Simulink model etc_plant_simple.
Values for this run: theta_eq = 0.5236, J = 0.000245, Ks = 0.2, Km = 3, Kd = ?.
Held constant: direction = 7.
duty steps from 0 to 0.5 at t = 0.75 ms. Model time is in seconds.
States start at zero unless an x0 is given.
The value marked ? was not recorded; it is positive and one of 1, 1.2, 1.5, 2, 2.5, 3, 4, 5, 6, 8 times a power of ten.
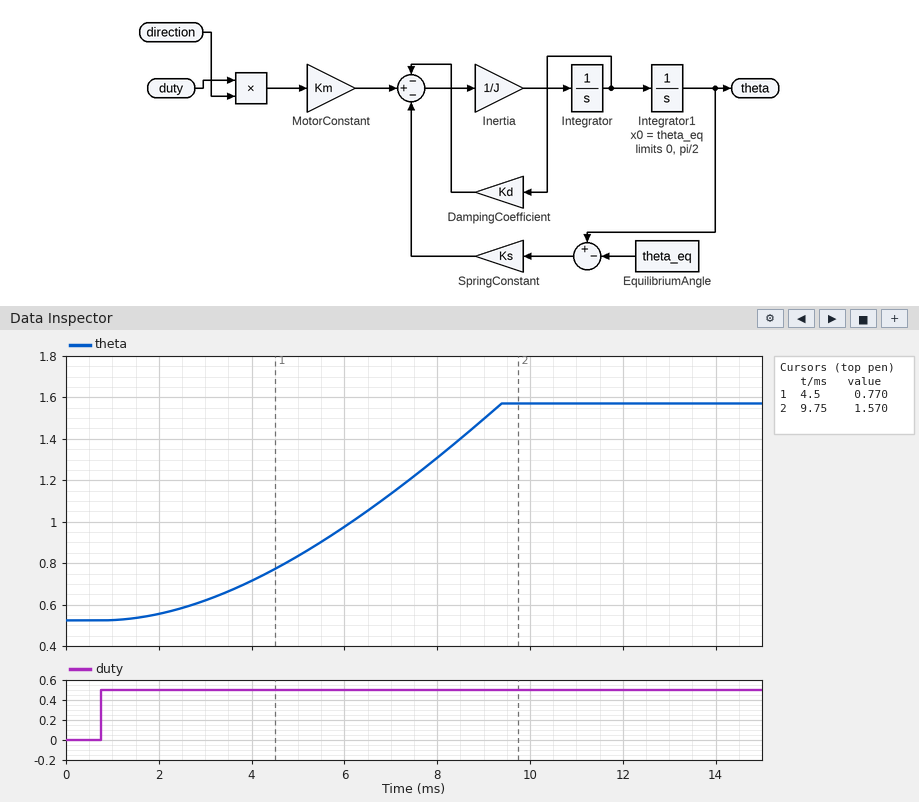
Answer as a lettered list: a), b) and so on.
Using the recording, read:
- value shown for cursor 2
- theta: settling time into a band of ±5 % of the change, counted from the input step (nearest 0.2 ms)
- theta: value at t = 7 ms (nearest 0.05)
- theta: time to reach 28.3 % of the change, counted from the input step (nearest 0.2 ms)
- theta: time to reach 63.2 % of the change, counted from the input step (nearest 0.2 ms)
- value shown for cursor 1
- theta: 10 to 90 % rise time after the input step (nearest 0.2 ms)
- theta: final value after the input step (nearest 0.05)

a) 1.570
b) 8.4 ms
c) 1.15
d) 4.2 ms
e) 6.6 ms
f) 0.770
g) 5.8 ms
h) 1.55
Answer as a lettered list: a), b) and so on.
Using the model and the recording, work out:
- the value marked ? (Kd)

a) 0.04
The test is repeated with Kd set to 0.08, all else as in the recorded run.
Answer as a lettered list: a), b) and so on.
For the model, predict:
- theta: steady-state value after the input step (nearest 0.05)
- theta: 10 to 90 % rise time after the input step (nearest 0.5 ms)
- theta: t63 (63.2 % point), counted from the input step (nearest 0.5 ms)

a) 1.55
b) 7.5 ms
c) 8.0 ms
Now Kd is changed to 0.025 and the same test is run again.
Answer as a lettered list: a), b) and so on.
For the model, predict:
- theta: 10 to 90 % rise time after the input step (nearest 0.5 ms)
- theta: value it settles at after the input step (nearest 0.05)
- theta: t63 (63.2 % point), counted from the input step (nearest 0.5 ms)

a) 5.0 ms
b) 1.55
c) 6.0 ms
